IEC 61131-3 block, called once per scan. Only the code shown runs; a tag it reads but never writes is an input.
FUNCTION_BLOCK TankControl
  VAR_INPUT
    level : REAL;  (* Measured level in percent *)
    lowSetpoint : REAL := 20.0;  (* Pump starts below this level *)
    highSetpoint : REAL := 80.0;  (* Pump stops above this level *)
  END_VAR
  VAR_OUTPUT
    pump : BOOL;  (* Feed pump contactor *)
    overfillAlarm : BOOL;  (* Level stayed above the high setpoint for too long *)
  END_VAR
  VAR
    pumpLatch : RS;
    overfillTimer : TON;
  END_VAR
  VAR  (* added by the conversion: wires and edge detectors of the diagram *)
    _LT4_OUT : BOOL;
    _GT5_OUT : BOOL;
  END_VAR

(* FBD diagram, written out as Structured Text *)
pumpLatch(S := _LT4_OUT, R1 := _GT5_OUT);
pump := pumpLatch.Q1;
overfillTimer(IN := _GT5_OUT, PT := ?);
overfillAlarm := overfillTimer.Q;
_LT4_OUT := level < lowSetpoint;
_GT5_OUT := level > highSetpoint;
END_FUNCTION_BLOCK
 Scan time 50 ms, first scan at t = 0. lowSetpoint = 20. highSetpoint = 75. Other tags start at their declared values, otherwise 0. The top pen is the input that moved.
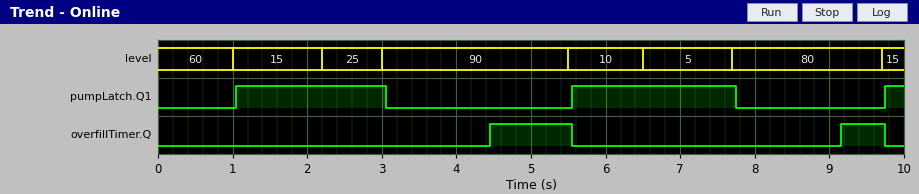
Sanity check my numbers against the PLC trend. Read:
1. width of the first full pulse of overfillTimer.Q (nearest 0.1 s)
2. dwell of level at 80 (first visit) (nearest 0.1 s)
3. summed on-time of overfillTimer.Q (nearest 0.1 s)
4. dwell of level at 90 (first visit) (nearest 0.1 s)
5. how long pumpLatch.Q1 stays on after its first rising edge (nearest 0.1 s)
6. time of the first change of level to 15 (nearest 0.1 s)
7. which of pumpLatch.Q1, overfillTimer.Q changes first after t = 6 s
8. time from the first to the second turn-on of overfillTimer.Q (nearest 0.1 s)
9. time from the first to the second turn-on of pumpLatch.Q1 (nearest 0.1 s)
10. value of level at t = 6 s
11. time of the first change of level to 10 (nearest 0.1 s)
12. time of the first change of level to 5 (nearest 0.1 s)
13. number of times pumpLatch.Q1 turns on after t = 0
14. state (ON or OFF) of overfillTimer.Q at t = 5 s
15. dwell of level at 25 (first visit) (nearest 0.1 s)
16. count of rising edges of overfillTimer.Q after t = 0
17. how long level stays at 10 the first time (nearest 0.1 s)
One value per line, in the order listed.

1.1 s
2.0 s
1.7 s
2.5 s
2.0 s
1.0 s
pumpLatch.Q1
4.7 s
4.5 s
10
5.5 s
6.5 s
3
ON
0.8 s
2
1.0 s
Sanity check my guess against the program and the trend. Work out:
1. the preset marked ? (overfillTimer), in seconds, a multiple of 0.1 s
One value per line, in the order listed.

1.4 s
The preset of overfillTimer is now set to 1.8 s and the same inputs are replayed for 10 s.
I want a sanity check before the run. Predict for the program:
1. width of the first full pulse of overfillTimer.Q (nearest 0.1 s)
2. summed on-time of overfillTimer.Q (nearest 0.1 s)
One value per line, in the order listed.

0.7 s
0.9 s
